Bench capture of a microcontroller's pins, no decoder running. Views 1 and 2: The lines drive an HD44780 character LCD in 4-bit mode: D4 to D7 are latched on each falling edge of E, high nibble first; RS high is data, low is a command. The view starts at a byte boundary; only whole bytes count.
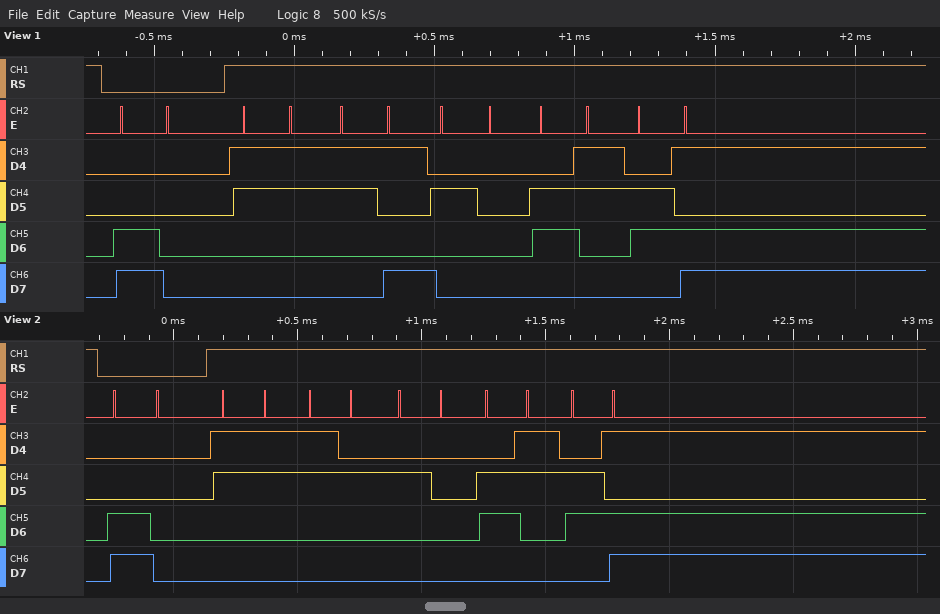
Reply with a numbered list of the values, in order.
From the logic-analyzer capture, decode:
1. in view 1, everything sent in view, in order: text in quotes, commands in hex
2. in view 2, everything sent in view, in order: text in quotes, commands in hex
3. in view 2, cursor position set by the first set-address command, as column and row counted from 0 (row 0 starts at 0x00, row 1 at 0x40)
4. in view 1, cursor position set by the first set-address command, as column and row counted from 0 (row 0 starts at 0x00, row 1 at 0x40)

1. 0xC0 "39 cm"
2. 0xC0 "32 cm"
3. column 0, row 1
4. column 0, row 1
